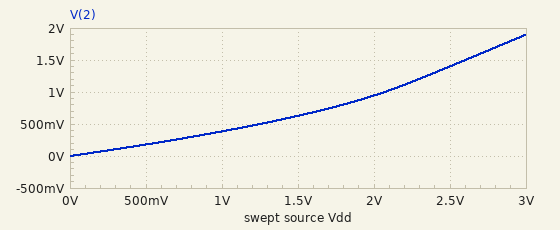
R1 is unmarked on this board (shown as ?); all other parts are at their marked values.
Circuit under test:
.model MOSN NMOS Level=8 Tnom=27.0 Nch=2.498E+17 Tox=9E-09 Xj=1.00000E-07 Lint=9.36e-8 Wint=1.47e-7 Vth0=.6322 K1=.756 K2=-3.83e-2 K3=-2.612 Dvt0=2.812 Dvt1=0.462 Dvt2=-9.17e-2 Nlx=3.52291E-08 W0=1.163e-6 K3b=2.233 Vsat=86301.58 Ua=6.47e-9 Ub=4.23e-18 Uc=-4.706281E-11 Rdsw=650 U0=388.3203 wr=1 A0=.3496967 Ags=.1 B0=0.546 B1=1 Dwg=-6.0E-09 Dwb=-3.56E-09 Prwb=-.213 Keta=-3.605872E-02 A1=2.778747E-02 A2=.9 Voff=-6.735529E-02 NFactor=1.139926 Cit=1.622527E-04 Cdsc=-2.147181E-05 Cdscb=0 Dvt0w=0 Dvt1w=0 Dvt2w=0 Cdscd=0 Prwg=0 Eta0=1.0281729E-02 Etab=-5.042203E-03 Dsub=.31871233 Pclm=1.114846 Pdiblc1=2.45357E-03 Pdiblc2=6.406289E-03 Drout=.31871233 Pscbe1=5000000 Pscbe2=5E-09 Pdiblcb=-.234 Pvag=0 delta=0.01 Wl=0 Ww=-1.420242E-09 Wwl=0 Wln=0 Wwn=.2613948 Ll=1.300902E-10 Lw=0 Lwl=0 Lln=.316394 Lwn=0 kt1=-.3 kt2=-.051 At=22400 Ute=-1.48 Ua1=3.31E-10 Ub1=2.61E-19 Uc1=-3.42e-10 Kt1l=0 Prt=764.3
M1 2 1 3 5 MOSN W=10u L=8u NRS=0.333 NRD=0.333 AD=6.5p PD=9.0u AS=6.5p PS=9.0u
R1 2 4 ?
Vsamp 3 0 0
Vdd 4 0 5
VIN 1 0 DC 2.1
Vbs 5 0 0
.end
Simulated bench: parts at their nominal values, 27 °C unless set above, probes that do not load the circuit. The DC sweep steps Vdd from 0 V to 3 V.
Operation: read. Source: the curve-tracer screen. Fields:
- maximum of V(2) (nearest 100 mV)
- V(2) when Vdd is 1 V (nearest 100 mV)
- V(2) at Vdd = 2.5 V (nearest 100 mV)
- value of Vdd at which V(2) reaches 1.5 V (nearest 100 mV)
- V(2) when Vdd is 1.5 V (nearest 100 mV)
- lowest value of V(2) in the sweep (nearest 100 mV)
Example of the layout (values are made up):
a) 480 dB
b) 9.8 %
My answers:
a) 1.9 V
b) 400 mV
c) 1.4 V
d) 2.6 V
e) 600 mV
f) 0 V
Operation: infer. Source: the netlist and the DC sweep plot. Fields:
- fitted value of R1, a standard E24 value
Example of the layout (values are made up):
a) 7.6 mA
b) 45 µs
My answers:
a) 24 kΩ
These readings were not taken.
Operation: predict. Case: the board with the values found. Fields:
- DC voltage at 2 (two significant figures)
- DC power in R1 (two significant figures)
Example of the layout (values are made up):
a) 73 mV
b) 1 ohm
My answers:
a) 3.9 V
b) 52 µW
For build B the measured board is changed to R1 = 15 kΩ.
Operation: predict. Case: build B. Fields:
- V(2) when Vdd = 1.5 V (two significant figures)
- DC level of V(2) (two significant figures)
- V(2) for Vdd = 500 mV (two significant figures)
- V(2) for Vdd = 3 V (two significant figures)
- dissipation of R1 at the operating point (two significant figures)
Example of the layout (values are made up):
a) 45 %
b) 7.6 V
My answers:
a) 860 mV
b) 4.3 V
c) 240 mV
d) 2.3 V
e) 33 µW
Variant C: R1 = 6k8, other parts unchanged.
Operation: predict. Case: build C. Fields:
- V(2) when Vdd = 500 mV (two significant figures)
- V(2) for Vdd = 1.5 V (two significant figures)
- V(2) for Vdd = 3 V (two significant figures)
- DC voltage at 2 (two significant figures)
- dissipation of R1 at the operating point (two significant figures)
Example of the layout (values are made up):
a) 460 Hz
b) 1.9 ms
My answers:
a) 340 mV
b) 1.2 V
c) 2.7 V
d) 4.7 V
e) 15 µW
